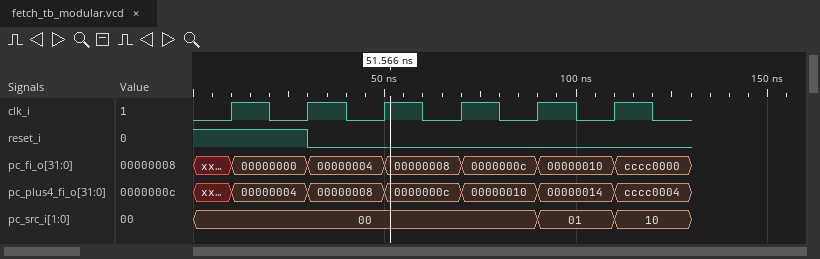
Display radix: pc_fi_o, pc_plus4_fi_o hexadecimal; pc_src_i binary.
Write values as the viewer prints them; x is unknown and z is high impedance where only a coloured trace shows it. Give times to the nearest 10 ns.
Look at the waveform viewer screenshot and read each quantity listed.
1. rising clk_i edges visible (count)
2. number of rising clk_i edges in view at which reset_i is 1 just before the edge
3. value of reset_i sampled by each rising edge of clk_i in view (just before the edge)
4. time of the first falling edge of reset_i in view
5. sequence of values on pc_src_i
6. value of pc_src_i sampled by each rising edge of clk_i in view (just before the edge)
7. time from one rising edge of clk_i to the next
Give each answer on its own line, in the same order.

6
2
1 1 0 0 0 0
30 ns
00, 01, 10
00, 00, 00, 00, 00, 01
20 ns
